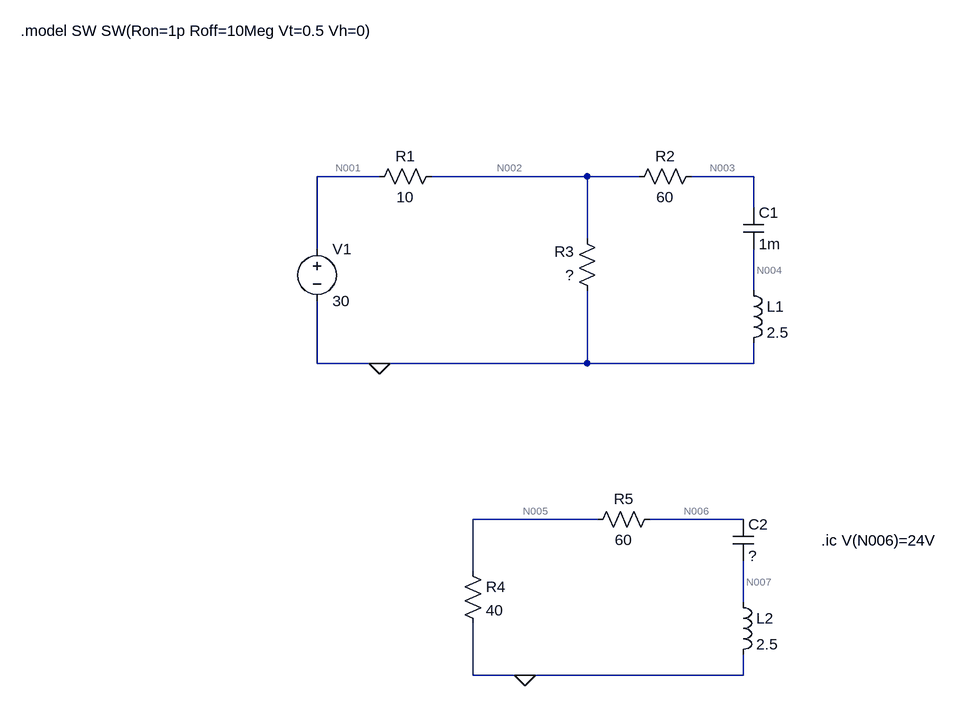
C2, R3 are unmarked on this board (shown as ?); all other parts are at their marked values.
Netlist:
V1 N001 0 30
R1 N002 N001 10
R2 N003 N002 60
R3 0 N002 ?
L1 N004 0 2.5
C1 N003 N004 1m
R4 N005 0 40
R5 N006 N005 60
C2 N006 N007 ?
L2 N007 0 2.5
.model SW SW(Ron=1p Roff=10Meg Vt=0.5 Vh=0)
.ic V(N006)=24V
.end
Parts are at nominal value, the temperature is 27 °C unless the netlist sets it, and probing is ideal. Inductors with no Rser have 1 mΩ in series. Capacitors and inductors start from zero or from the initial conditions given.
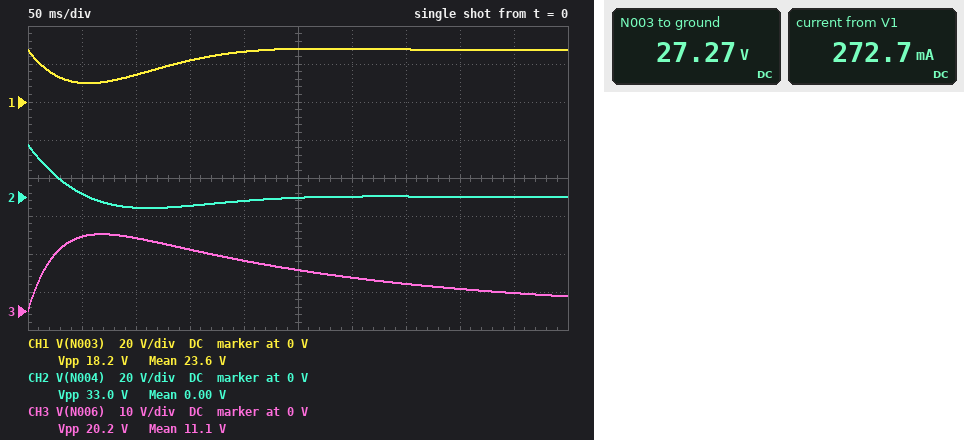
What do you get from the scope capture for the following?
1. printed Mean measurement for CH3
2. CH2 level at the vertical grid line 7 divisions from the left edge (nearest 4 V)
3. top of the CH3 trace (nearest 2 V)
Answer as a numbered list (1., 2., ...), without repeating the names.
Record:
1. 11.1 V
2. 0 V
3. 20 V
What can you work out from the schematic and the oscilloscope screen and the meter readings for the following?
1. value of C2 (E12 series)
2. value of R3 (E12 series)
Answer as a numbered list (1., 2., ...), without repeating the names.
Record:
1. 2.7 mF
2. 100 Ω
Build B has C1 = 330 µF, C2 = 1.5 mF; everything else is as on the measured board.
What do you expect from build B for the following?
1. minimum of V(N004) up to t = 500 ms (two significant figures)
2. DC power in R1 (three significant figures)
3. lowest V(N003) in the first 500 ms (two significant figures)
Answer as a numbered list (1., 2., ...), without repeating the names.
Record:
1. -10 V
2. 744 mW
3. 14 V
